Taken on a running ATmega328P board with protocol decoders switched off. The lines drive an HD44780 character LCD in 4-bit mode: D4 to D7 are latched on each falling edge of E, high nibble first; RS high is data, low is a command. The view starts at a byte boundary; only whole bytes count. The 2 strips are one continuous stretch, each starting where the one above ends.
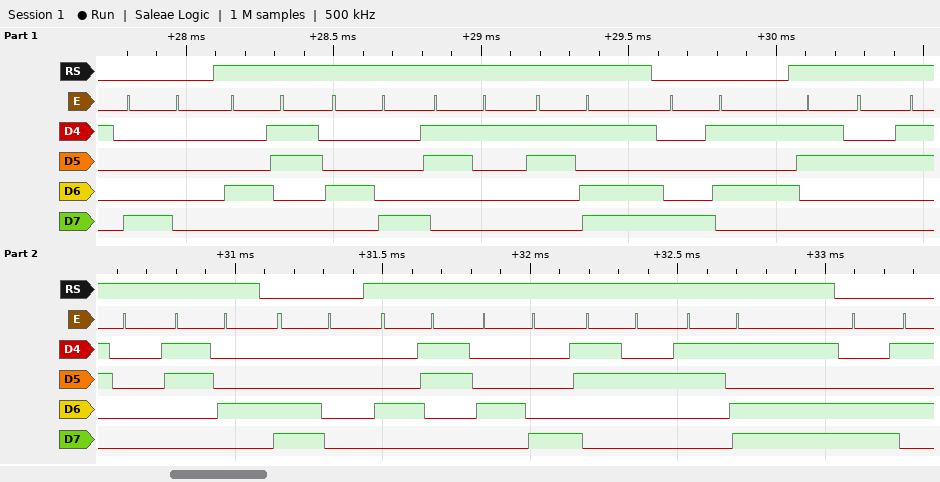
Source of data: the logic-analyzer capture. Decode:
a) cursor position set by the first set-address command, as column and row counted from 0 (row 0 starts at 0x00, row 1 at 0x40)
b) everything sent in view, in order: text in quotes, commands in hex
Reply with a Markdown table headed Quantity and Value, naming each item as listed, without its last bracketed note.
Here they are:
| Quantity | Value |
|---|---|
| cursor position set by the first set-address command, as column and row counted from 0 | column 0, row 0 |
| everything sent in view, in order: text in quotes, commands in hex | 0x80 "CH1=" 0x85 "204" 0xC0 "CH2=" 0xC5 |
